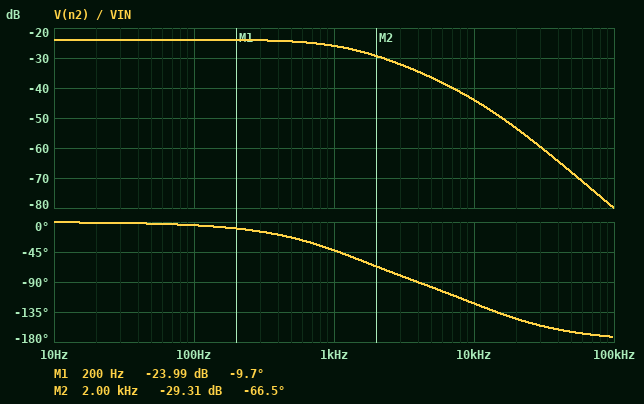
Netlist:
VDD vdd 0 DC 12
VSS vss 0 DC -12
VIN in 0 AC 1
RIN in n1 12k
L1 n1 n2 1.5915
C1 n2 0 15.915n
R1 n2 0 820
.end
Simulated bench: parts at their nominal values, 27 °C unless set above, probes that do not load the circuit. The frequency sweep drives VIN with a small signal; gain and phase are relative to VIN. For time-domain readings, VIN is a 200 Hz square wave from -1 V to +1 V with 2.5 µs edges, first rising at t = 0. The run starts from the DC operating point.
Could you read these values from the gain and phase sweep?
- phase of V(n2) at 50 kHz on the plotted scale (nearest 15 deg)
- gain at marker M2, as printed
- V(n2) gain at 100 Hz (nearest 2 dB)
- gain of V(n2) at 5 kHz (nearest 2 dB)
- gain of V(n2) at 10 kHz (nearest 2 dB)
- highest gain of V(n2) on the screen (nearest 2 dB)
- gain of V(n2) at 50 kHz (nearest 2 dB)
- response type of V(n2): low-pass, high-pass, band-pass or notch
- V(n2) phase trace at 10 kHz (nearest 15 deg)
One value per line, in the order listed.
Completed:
-165 deg
-29.31 dB
-24 dB
-36 dB
-44 dB
-24 dB
-68 dB
low-pass
-120 deg
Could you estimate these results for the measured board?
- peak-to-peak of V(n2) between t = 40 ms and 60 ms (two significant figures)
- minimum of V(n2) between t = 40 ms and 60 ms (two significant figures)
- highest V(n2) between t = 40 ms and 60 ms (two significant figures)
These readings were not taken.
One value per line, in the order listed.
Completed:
130 mV
-64 mV
64 mV
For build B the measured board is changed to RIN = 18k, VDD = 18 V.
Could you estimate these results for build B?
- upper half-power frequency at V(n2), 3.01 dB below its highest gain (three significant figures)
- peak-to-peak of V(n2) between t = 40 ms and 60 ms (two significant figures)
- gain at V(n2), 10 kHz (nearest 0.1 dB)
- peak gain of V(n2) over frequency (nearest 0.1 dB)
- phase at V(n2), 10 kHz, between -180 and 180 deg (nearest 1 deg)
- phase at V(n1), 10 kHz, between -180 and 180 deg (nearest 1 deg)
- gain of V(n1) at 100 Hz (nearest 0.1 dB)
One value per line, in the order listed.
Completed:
1.85 kHz
87 mV
-44.1 dB
-27.2 dB
-119 deg
10 deg
-23.3 dB
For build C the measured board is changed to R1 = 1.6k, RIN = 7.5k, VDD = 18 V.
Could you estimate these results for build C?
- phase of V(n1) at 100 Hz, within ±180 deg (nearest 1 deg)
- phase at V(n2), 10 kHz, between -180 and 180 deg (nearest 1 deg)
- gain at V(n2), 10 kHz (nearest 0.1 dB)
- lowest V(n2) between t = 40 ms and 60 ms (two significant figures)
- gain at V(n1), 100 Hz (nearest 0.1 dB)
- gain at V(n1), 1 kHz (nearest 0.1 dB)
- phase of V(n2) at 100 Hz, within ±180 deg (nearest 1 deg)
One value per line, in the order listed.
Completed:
25 deg
-143 deg
-41.4 dB
-180 mV
-13.8 dB
-2.6 dB
-7 deg
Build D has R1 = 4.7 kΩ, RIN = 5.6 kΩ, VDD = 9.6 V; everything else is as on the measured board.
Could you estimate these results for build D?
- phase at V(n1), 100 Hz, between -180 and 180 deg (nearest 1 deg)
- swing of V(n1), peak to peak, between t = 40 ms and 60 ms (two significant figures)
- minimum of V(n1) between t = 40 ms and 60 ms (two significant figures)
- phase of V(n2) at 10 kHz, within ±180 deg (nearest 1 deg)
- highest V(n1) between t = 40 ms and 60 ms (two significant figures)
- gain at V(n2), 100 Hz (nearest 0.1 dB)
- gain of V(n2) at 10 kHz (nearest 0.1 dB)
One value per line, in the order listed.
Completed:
5 deg
3.1 V
-1.5 V
-165 deg
1.5 V
-6.8 dB
-40.1 dB
